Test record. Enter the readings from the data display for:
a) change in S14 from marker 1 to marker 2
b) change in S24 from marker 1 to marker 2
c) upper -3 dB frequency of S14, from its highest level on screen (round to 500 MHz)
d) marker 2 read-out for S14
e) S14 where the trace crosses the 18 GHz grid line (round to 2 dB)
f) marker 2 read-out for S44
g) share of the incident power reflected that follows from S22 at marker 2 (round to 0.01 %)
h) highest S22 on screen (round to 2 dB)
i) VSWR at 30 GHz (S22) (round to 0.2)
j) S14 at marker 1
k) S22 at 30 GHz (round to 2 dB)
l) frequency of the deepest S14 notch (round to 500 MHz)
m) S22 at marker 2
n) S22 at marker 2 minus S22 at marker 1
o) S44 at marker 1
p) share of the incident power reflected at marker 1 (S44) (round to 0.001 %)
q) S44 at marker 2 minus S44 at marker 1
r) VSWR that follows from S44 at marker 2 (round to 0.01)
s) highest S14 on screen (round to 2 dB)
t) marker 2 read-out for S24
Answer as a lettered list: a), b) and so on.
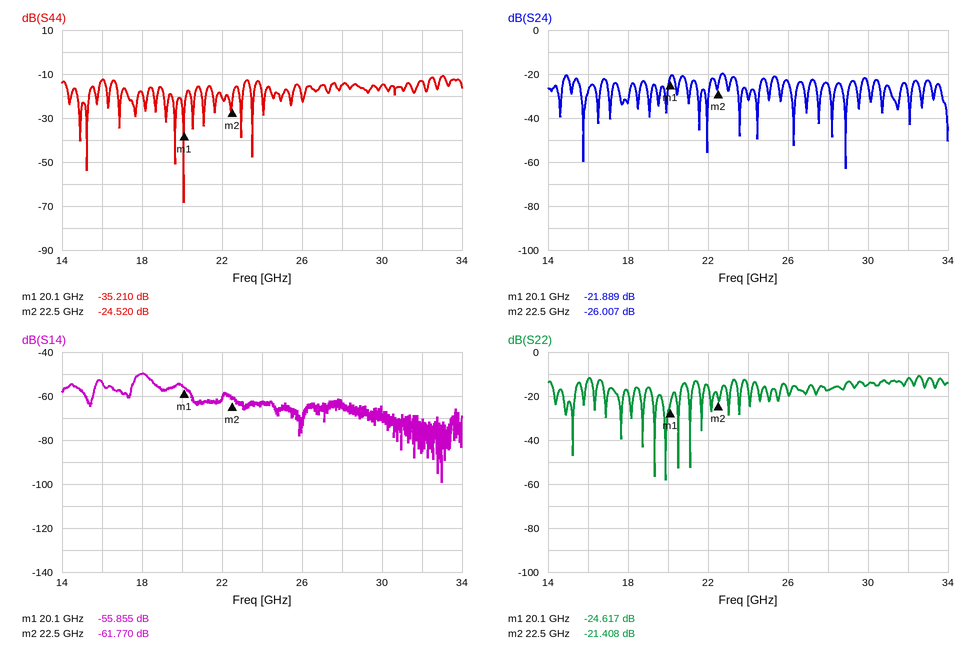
a) -5.915 dB
b) -4.118 dB
c) 18.5 GHz
d) -61.770 dB
e) -50 dB
f) -24.520 dB
g) 0.72 %
h) -10 dB
i) 1.4
j) -55.855 dB
k) -14 dB
l) 33.0 GHz
m) -21.408 dB
n) 3.209 dB
o) -35.210 dB
p) 0.030 %
q) 10.690 dB
r) 1.13
s) -50 dB
t) -26.007 dB
